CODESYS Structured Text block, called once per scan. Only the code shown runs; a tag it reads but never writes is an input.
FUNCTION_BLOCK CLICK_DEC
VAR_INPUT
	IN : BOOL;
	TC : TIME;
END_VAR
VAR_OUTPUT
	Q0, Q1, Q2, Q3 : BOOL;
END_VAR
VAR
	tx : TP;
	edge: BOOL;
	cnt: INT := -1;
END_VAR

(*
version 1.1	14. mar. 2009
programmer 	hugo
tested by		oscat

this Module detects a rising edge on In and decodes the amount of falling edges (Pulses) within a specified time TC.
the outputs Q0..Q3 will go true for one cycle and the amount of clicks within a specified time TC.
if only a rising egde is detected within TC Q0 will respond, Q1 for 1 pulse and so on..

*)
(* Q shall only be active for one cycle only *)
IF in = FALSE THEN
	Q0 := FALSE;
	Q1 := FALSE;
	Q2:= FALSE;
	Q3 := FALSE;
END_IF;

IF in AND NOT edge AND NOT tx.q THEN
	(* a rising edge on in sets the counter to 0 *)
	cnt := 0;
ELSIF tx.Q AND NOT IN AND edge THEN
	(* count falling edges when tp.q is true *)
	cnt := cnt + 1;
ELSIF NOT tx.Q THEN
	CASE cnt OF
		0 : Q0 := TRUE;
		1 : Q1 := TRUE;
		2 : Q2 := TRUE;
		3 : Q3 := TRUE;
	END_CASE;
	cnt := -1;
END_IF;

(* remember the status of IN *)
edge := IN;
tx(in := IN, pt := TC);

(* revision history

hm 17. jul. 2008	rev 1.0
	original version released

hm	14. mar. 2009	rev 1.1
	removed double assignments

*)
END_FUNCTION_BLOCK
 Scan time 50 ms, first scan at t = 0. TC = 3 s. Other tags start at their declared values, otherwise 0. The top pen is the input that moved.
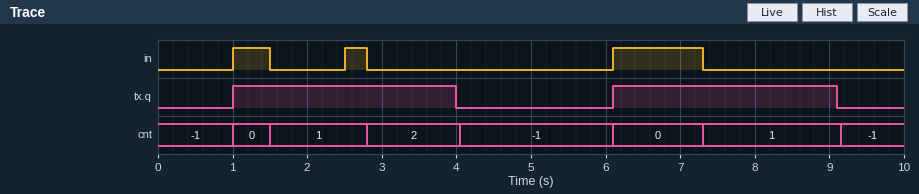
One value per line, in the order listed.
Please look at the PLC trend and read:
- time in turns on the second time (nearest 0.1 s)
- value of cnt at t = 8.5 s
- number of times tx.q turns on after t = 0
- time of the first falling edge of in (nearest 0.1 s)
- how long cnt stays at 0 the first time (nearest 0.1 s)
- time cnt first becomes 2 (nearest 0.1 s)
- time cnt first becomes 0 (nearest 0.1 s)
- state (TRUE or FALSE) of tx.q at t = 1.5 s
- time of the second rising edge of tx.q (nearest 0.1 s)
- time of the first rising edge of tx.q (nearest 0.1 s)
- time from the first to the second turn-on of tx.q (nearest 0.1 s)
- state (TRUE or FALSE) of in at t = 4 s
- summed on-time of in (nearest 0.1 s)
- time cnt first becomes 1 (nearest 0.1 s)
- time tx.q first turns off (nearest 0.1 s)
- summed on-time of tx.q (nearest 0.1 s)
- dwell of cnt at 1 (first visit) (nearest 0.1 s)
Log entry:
2.5 s
1
2
1.5 s
0.5 s
2.8 s
1.0 s
TRUE
6.1 s
1.0 s
5.1 s
FALSE
2.0 s
1.5 s
4.0 s
6.0 s
1.3 s
